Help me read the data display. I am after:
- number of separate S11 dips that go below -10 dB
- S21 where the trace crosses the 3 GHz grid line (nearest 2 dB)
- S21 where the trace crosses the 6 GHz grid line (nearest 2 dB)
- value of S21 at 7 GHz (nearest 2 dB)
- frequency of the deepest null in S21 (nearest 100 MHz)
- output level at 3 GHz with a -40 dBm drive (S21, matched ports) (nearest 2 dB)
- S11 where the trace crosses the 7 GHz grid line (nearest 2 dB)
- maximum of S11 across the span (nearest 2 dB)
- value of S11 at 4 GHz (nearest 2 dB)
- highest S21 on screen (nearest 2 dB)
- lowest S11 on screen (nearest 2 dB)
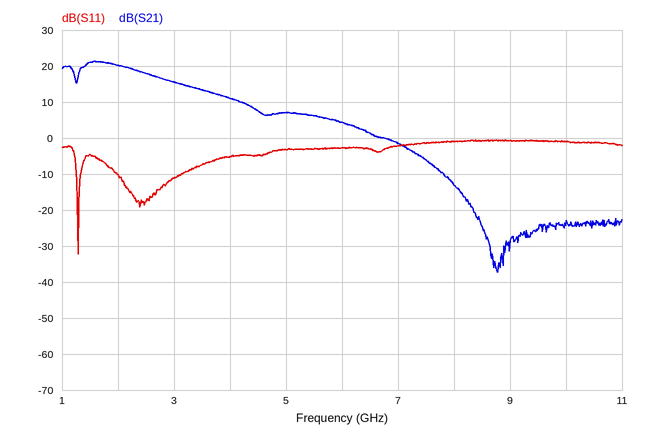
2
16 dB
4 dB
-2 dB
8.8 GHz
-24 dBm
-2 dB
0 dB
-6 dB
22 dB
-32 dB
